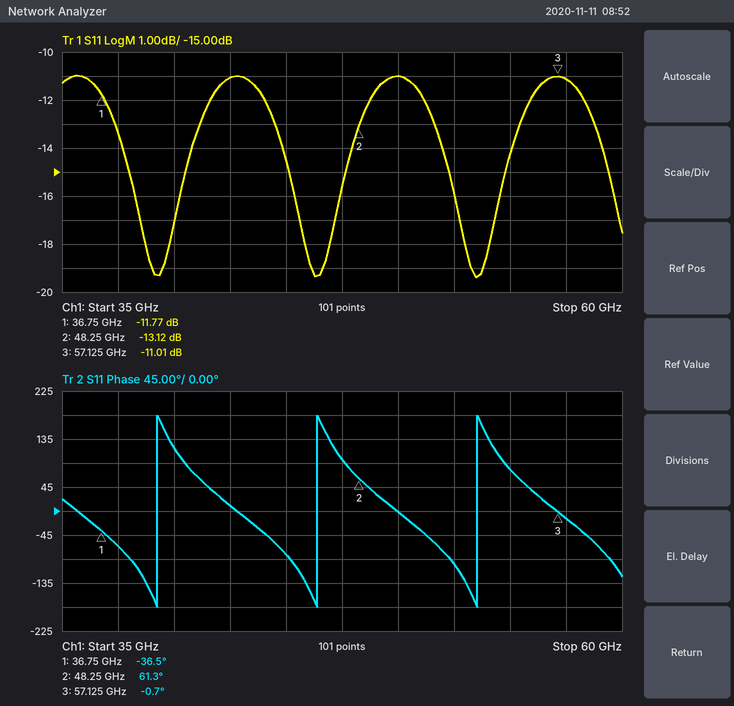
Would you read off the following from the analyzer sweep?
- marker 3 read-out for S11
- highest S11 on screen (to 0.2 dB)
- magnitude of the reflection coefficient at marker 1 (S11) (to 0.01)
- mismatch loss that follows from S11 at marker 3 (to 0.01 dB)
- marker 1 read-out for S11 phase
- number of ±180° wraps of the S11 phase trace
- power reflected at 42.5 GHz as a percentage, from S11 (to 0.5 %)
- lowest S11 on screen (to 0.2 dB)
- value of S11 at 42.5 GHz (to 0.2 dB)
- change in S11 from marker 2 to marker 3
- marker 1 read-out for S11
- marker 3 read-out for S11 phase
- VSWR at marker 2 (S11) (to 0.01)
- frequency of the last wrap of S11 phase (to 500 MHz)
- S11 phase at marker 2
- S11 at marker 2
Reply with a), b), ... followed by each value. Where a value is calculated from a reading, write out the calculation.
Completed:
a) -11.01 dB
b) -11.0 dB
c) 10^(-11.77/20) ≈ 0.26
d) −10 log10(1 − 10^(-11.01/10)) ≈ 0.36 dB
e) -36.5°
f) 3
g) 10^(-11/10) ≈ 7.94 %, so 8.0 % to the nearest 0.5 %
h) -19.4 dB
i) -11.0 dB
j) -11.01 − (-13.12) = 2.11 dB
k) -11.77 dB
l) -0.7°
m) (1 + 0.2208)/(1 − 0.2208) ≈ 1.57
n) 53.5 GHz
o) 61.3°
p) -13.12 dB
